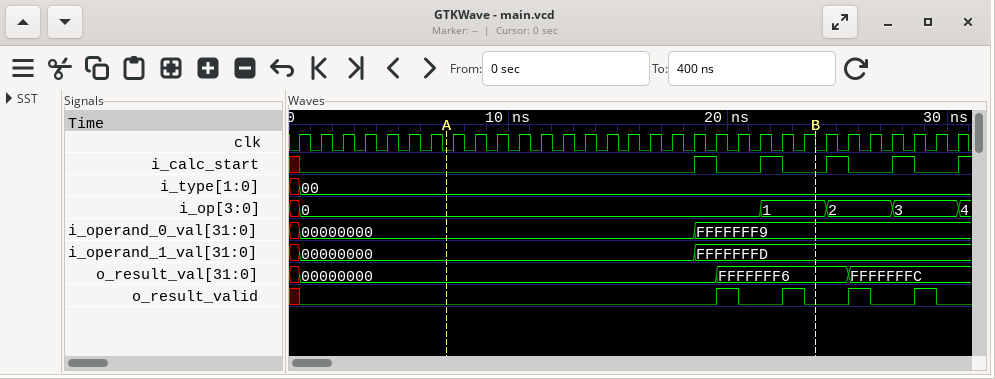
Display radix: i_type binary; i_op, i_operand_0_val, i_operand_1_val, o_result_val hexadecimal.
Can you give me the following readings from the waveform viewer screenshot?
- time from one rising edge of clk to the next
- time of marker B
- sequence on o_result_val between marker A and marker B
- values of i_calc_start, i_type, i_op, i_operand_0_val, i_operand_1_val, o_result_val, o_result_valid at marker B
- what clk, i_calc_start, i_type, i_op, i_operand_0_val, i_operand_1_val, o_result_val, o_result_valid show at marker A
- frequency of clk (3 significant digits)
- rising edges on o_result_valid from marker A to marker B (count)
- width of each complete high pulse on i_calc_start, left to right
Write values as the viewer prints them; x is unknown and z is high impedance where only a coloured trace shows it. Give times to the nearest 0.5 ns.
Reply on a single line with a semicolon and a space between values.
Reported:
1 ns; 24 ns; 00000000, FFFFFFF6; i_calc_start=0, i_type=00, i_op=1, i_operand_0_val=FFFFFFF9, i_operand_1_val=FFFFFFFD, o_result_val=FFFFFFF6, o_result_valid=0; clk=0, i_calc_start=0, i_type=00, i_op=0, i_operand_0_val=00000000, i_operand_1_val=00000000, o_result_val=00000000, o_result_valid=0; 1.00 GHz; 2; 1 ns, 1 ns, 1 ns, 1 ns
